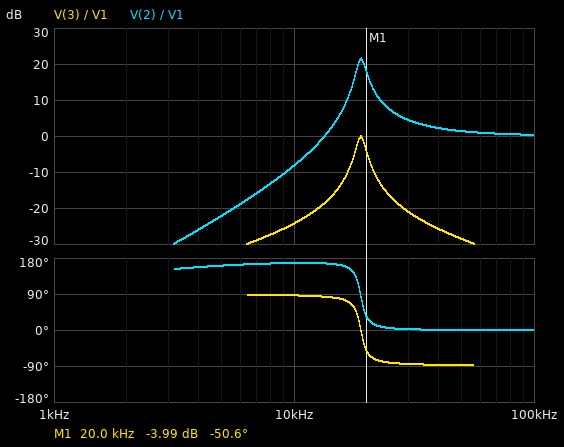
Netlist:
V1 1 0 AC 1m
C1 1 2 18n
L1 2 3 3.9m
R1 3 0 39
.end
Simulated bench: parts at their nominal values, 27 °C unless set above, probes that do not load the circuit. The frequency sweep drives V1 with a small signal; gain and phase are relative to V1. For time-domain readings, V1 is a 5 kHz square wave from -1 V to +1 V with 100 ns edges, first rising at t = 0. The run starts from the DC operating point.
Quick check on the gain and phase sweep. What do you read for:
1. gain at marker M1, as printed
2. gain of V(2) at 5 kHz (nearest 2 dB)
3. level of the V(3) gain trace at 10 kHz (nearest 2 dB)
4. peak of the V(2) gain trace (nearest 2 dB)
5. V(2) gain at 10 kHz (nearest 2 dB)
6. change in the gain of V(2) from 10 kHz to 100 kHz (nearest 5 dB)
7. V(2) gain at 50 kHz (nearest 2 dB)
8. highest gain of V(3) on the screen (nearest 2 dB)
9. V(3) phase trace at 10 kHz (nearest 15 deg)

-3.99 dB
-22 dB
-24 dB
22 dB
-8 dB
10 dB
2 dB
0 dB
90 deg
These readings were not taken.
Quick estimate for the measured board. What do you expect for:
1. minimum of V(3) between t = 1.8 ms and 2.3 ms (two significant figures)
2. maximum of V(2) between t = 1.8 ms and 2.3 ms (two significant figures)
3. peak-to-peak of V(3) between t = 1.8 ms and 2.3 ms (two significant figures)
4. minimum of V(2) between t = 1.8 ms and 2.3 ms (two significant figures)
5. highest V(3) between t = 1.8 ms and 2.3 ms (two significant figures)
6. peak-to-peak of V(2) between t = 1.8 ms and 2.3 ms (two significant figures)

-100 mV
1.3 V
210 mV
-1.3 V
100 mV
2.6 V
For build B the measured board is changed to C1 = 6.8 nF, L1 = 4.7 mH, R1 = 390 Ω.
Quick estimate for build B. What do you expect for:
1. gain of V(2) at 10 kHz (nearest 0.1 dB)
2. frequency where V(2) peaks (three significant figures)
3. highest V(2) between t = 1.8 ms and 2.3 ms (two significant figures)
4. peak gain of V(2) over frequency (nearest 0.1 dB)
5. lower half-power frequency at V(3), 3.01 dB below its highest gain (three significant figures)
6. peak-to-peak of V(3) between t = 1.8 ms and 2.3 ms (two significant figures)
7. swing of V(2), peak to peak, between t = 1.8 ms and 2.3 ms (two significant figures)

-12.6 dB
29.5 kHz
2.0 V
7.6 dB
22.3 kHz
1.4 V
4.0 V
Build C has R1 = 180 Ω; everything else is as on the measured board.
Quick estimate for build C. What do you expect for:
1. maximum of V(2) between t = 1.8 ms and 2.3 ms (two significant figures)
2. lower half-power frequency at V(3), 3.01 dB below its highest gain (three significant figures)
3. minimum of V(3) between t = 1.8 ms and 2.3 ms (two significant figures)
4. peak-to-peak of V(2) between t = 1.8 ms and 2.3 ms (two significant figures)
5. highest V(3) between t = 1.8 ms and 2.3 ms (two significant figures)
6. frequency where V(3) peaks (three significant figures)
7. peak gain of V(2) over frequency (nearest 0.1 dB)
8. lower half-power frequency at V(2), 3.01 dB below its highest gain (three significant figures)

1.9 V
15.7 kHz
-560 mV
3.8 V
560 mV
19.0 kHz
9.0 dB
16.5 kHz
